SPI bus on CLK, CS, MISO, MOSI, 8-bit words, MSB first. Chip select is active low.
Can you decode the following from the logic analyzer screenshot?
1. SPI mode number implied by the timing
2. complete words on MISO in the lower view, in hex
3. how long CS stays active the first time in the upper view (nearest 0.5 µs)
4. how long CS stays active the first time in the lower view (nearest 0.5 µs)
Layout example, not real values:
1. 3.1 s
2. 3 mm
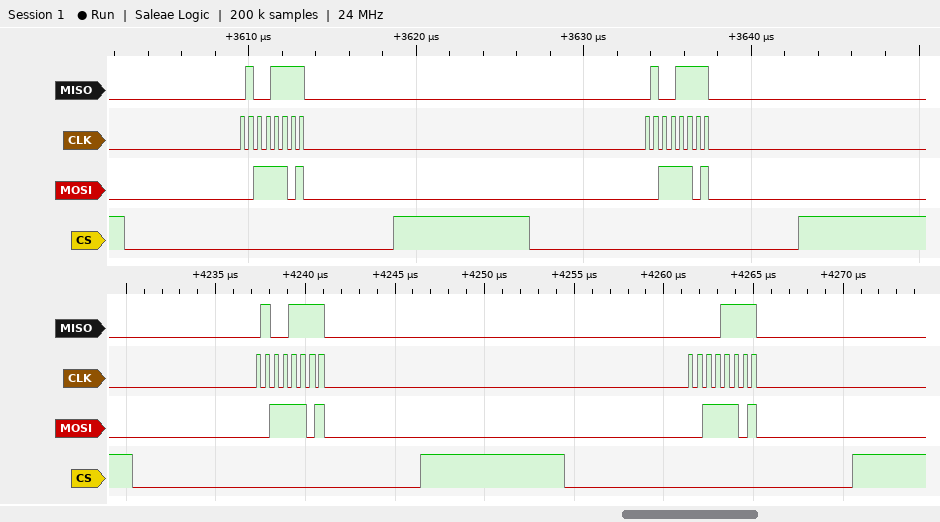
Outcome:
1. 0
2. 4F, 0F
3. 16 µs
4. 16 µs
